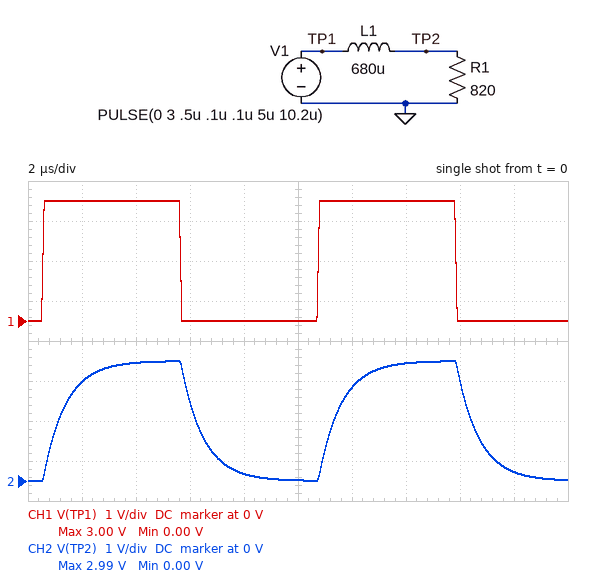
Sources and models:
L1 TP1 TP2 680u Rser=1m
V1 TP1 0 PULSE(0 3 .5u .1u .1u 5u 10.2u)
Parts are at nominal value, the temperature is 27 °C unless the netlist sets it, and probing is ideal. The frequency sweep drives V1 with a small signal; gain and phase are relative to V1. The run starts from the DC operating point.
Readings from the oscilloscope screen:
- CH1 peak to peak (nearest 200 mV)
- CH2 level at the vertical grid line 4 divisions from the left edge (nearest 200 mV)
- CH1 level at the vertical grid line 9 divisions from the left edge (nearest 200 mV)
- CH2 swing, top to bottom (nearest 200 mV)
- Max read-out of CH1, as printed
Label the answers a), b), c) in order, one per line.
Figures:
a) 3.0 V
b) 200 mV
c) 0 V
d) 3.0 V
e) 3.00 V
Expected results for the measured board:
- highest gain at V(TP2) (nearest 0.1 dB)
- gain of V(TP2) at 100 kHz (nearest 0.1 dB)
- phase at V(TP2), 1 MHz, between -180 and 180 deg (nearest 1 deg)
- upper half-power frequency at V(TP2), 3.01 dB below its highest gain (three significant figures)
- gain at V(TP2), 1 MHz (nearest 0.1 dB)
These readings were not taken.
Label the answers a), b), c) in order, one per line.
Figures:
a) 0 dB
b) -1.0 dB
c) -79 deg
d) 192 kHz
e) -14.5 dB
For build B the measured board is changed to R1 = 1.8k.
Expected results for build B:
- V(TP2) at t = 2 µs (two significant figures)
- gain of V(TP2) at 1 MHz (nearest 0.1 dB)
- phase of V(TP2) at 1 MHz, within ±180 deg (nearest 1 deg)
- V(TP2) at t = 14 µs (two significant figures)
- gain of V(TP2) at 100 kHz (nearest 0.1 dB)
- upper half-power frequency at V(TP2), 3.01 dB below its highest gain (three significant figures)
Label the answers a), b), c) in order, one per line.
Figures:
a) 2.9 V
b) -8.2 dB
c) -67 deg
d) 3.0 V
e) -0.2 dB
f) 421 kHz
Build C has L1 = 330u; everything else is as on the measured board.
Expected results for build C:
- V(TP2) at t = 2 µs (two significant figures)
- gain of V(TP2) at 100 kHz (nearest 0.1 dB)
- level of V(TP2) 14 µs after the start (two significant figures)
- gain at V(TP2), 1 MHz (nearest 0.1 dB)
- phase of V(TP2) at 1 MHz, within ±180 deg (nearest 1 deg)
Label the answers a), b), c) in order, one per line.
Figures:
a) 2.9 V
b) -0.3 dB
c) 3.0 V
d) -8.7 dB
e) -68 deg
